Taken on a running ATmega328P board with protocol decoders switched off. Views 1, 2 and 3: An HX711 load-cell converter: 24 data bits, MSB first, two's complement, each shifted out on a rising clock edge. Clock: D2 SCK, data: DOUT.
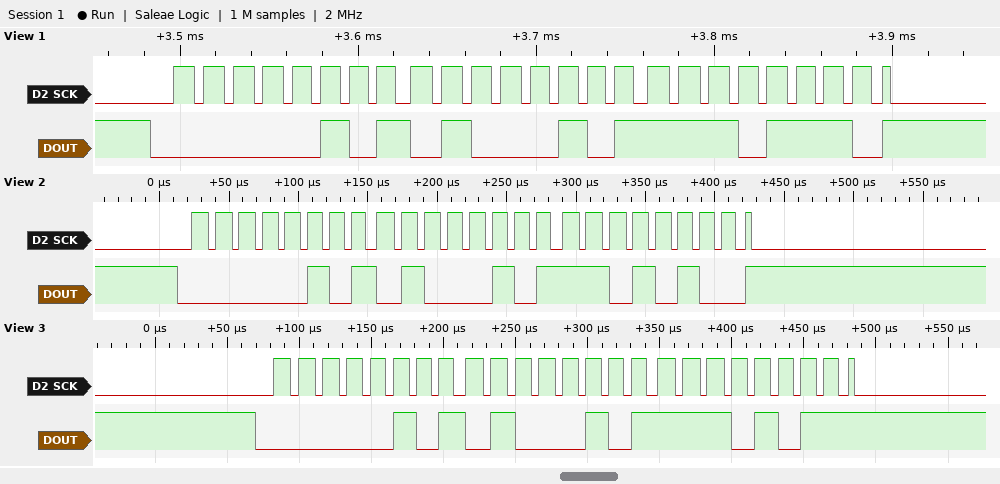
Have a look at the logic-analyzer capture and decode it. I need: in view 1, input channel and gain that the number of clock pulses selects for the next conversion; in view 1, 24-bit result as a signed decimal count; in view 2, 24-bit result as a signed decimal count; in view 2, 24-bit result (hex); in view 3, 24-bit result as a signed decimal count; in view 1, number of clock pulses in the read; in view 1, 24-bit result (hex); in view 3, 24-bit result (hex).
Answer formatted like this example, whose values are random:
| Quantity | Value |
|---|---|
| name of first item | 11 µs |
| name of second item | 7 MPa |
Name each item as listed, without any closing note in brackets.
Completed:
| Quantity | Value |
|---|---|
| in view 1, input channel and gain that the number of clock pulses selects for the next conversion | channel A, gain 128 |
| in view 1, 24-bit result as a signed decimal count | 345582 |
| in view 2, 24-bit result as a signed decimal count | 345556 |
| in view 2, 24-bit result | 0x0545D4 |
| in view 3, 24-bit result as a signed decimal count | 345579 |
| in view 1, number of clock pulses in the read | 25 |
| in view 1, 24-bit result | 0x0545EE |
| in view 3, 24-bit result | 0x0545EB |
